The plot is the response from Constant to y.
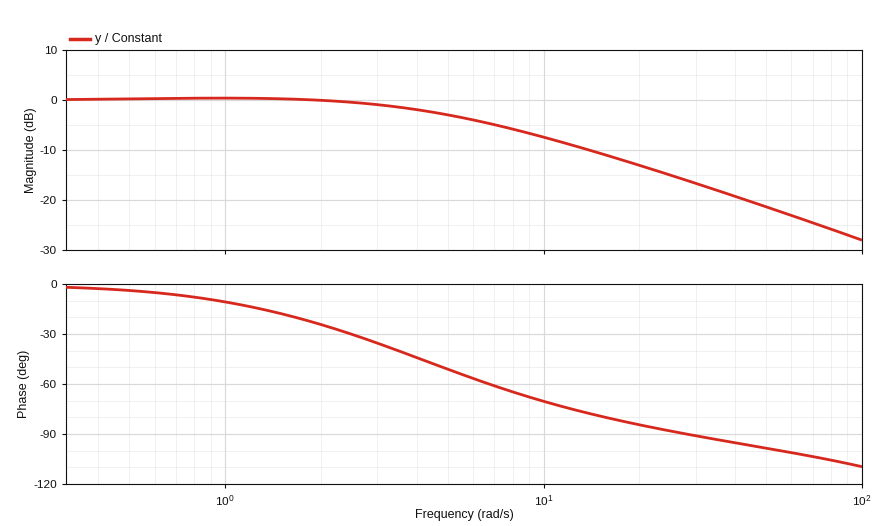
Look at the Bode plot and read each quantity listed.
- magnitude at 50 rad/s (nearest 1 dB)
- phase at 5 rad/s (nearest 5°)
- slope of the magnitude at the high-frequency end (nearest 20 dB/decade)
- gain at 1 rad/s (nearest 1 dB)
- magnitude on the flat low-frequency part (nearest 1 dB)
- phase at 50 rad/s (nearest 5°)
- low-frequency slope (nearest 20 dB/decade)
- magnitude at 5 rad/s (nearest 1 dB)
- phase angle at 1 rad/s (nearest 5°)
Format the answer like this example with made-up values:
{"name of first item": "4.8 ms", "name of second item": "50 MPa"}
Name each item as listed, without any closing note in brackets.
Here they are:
{"magnitude at 50 rad/s": "-21 dB", "phase at 5 rad/s": "-50°", "slope of the magnitude at the high-frequency end": "-20 dB/decade", "gain at 1 rad/s": "0 dB", "magnitude on the flat low-frequency part": "0 dB", "phase at 50 rad/s": "-100°", "low-frequency slope": "0 dB/decade", "magnitude at 5 rad/s": "-3 dB", "phase angle at 1 rad/s": "-10°"}
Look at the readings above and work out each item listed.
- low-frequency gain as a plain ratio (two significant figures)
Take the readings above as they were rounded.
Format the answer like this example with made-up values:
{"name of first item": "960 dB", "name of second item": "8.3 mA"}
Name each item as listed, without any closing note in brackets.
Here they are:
{"low-frequency gain as a plain ratio": "1.0"}
